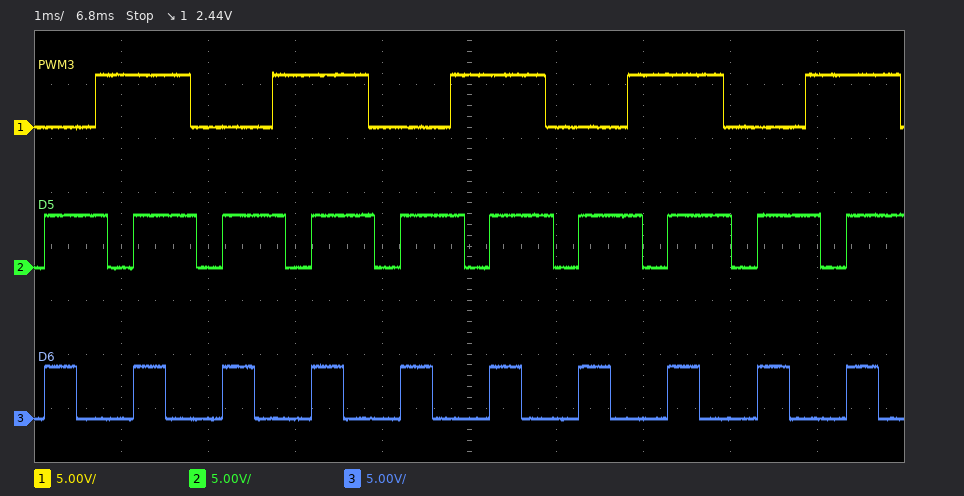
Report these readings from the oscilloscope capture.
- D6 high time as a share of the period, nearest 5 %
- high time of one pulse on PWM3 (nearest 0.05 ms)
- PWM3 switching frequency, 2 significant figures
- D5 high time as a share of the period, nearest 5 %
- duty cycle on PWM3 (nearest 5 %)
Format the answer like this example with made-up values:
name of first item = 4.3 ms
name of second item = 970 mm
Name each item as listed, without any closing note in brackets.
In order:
D6 high time as a share of the period, nearest 5 % = 35 %
high time of one pulse on PWM3 = 1.10 ms
PWM3 switching frequency, 2 significant figures = 490 Hz
D5 high time as a share of the period, nearest 5 % = 70 %
duty cycle on PWM3 = 55 %
